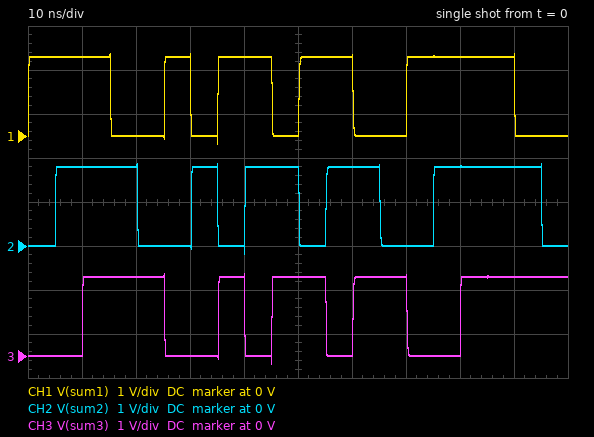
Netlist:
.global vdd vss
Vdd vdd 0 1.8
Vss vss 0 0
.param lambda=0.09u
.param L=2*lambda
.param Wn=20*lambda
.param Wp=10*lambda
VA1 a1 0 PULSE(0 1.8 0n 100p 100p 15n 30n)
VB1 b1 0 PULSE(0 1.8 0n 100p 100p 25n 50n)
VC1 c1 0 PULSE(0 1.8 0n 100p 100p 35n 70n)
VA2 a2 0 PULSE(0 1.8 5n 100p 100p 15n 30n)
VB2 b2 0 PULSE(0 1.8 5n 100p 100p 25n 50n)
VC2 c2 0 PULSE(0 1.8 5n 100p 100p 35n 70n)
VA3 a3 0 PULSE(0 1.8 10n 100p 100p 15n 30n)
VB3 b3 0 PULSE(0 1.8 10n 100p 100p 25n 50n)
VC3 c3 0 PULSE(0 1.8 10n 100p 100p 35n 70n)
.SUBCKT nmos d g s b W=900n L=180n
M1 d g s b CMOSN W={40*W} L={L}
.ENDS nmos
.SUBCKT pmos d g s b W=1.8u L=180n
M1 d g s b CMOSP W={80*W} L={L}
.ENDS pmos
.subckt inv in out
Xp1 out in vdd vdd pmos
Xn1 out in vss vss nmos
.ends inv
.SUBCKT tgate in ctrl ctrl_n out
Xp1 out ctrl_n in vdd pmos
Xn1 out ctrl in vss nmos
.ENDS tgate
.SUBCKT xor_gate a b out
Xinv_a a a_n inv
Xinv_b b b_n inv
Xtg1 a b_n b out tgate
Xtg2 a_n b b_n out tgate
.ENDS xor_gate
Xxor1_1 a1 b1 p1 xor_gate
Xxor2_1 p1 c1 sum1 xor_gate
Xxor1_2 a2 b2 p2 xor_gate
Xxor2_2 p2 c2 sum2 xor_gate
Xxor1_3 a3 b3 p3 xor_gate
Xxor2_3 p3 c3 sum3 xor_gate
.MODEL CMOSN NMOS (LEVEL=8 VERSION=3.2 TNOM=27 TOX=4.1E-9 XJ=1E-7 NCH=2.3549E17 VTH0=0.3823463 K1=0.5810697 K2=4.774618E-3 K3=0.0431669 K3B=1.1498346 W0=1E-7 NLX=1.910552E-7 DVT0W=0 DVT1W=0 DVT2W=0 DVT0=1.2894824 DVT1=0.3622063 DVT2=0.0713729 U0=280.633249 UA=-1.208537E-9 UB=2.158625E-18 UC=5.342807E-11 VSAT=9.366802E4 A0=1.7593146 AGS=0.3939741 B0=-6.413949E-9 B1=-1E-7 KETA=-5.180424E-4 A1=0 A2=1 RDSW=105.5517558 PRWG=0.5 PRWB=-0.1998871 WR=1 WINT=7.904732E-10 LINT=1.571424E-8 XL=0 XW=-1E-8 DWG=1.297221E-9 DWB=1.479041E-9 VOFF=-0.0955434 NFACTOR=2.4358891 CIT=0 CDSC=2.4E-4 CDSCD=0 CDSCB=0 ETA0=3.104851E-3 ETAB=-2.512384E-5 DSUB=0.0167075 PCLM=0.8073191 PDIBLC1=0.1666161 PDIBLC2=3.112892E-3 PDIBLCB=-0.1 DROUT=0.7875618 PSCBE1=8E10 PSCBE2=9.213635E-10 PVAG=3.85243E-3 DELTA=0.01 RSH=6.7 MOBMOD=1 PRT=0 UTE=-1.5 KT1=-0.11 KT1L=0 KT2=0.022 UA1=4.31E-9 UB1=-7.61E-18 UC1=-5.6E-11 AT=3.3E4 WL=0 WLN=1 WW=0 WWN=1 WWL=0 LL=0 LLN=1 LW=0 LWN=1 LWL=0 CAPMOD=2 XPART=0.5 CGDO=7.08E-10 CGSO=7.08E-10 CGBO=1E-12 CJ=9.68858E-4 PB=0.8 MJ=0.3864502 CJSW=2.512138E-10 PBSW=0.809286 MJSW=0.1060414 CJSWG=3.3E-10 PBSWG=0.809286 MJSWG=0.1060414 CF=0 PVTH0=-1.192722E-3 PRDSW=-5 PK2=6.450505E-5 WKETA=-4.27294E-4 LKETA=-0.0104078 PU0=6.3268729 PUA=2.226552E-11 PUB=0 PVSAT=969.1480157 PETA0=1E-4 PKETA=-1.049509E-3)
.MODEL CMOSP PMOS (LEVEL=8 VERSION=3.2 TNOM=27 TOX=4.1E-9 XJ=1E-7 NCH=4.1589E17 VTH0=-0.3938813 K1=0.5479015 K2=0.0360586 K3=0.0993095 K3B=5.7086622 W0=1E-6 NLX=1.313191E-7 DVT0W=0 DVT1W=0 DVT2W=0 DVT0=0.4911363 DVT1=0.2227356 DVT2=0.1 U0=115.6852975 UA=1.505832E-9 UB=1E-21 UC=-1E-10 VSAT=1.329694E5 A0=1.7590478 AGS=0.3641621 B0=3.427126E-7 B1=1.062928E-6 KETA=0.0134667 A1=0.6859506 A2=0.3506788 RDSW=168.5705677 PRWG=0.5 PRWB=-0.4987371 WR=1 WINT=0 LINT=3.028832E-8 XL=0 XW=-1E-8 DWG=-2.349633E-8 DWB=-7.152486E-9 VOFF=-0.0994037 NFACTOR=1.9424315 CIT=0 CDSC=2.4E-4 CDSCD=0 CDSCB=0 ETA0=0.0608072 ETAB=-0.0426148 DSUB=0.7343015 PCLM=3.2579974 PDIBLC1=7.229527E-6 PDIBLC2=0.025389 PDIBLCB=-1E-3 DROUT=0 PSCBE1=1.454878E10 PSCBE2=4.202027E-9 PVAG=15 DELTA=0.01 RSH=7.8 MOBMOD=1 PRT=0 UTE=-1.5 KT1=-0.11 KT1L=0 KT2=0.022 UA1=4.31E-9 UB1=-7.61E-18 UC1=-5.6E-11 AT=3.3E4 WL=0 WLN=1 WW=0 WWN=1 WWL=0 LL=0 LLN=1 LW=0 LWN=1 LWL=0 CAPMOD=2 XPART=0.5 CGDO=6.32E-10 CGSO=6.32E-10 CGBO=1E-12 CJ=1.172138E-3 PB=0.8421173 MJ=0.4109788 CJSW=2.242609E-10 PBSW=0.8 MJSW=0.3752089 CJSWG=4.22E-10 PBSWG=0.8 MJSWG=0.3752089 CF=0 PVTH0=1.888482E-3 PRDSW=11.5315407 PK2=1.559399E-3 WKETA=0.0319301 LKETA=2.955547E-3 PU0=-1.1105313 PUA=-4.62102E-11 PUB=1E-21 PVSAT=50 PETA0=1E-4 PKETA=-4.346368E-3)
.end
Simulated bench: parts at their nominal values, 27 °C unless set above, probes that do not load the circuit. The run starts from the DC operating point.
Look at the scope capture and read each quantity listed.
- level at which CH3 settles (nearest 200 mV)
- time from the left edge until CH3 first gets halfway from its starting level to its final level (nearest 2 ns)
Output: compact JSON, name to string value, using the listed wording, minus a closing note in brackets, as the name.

{"level at which CH3 settles": "1.8 V", "time from the left edge until CH3 first gets halfway from its starting level to its final level": "10 ns"}
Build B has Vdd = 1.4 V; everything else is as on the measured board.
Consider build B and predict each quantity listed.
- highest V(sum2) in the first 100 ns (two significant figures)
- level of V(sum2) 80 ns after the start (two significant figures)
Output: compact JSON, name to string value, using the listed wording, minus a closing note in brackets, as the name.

{"highest V(sum2) in the first 100 ns": "1.8 V", "level of V(sum2) 80 ns after the start": "1.4 V"}
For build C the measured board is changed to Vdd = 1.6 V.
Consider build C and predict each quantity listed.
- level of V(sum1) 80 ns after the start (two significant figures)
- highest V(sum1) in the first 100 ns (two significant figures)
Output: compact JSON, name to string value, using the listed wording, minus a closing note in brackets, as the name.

{"level of V(sum1) 80 ns after the start": "1.6 V", "highest V(sum1) in the first 100 ns": "1.8 V"}
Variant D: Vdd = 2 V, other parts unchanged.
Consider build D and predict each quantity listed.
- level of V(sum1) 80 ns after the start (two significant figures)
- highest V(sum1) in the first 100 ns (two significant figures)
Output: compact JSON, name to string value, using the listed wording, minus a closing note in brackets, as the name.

{"level of V(sum1) 80 ns after the start": "2.0 V", "highest V(sum1) in the first 100 ns": "2.1 V"}
